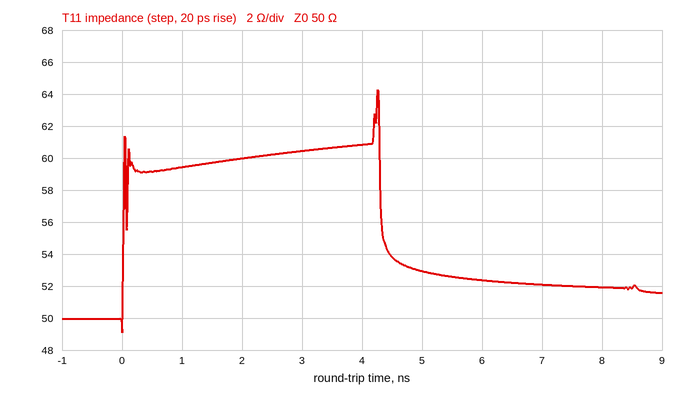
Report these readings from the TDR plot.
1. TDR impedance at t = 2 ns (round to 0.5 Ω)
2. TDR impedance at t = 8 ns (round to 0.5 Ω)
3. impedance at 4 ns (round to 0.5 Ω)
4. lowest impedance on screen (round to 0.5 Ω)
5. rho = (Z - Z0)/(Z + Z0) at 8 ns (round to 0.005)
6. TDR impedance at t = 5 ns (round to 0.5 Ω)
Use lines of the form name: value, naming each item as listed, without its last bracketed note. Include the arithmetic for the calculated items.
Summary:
TDR impedance at t = 2 ns: 60.0 Ω
TDR impedance at t = 8 ns: 52.0 Ω
impedance at 4 ns: 61.0 Ω
lowest impedance on screen: 49.0 Ω
rho = (Z - Z0)/(Z + Z0) at 8 ns: (52 − 50)/(52 + 50) ≈ +0.020
TDR impedance at t = 5 ns: 53.0 Ω
